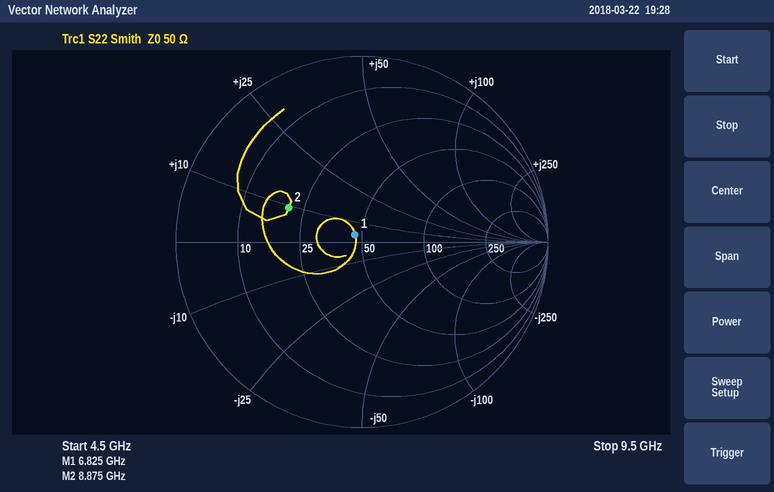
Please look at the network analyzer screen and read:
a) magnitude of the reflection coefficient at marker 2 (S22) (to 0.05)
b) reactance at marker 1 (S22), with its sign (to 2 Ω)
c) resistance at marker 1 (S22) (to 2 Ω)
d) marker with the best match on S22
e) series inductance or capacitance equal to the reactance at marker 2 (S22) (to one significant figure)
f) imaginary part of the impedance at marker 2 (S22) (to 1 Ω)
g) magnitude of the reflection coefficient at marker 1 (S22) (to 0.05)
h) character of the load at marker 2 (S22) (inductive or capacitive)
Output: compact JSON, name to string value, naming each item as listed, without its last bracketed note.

{"magnitude of the reflection coefficient at marker 2 (S22)": "0.45", "reactance at marker 1 (S22), with its sign": "+4 Ω", "resistance at marker 1 (S22)": "46 Ω", "marker with the best match on S22": "marker 1", "series inductance or capacitance equal to the reactance at marker 2 (S22)": "200 pH", "imaginary part of the impedance at marker 2 (S22)": "+9 Ω", "magnitude of the reflection coefficient at marker 1 (S22)": "0.05", "character of the load at marker 2 (S22)": "inductive"}
